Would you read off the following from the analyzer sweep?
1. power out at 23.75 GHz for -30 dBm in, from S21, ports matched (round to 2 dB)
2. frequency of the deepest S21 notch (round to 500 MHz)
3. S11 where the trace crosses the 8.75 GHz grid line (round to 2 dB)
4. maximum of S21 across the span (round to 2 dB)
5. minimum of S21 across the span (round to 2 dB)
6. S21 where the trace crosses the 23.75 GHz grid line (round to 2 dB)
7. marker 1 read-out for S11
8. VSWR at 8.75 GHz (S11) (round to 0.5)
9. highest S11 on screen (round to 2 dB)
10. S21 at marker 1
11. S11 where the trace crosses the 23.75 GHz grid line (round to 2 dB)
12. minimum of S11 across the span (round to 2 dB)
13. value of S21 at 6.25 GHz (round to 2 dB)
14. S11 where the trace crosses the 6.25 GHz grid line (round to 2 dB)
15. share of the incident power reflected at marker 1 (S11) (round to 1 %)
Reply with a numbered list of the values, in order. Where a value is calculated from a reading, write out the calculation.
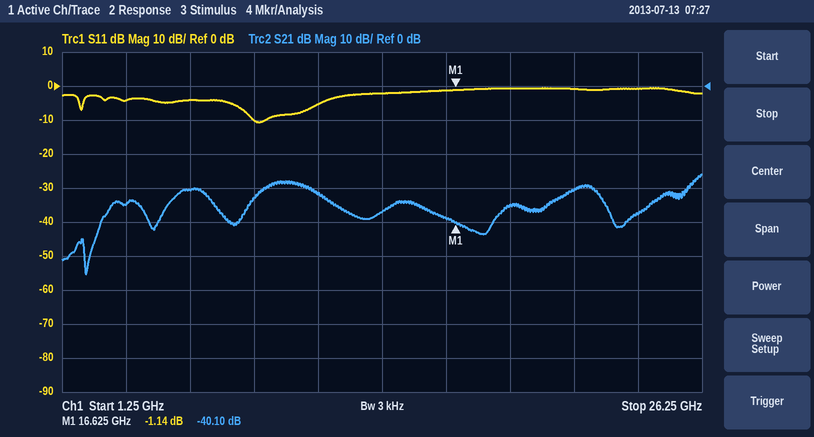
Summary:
1. -30 dBm + (-38 dB) = -68 dBm
2. 2.0 GHz
3. -10 dB
4. -26 dB
5. -56 dB
6. -38 dB
7. -1.14 dB
8. |Γ| = 10^(-10/20) = 0.3162; VSWR = (1 + 0.3162)/(1 − 0.3162) ≈ 1.92, so 2.0 to the nearest 0.5
9. 0 dB
10. -40.10 dB
11. 0 dB
12. -10 dB
13. -30 dB
14. -4 dB
15. 10^(-1.14/10) ≈ 77 %
